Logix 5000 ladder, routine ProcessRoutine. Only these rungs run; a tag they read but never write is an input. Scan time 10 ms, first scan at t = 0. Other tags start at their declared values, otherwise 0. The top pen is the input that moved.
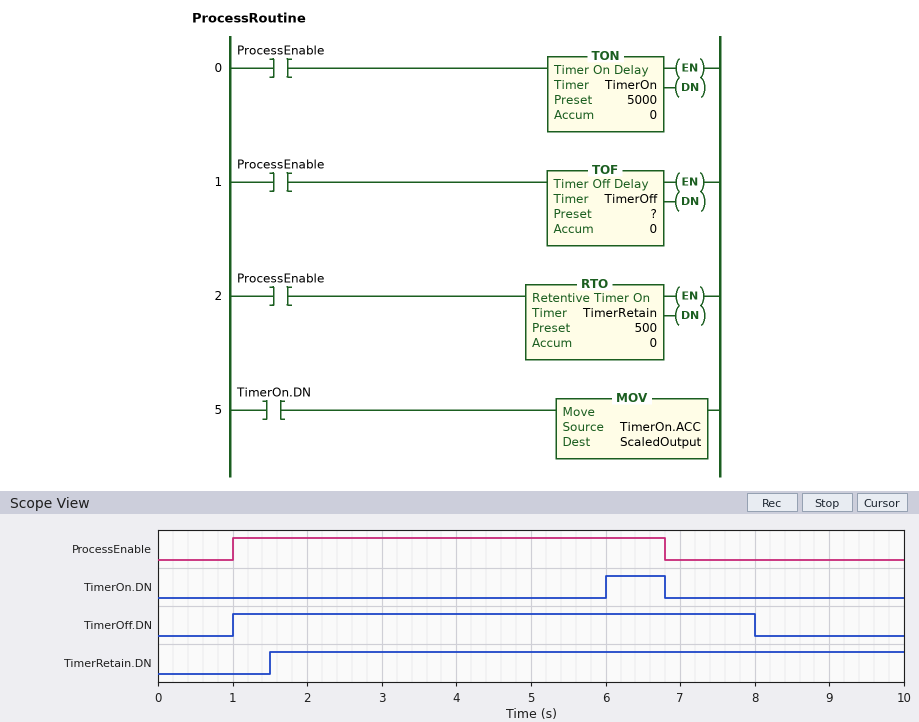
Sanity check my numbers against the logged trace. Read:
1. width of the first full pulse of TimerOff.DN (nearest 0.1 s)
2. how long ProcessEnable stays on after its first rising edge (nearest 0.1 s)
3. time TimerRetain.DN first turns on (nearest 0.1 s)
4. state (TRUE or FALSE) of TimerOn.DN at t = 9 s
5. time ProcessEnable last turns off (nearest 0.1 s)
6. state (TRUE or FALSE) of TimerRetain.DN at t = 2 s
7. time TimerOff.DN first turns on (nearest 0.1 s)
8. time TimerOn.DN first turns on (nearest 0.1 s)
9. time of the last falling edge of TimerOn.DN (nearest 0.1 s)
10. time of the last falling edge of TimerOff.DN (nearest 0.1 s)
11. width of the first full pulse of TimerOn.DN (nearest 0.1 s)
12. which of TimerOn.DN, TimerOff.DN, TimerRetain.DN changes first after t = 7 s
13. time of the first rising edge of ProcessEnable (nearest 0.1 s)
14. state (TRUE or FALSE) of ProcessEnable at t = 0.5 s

7.0 s
5.8 s
1.5 s
FALSE
6.8 s
TRUE
1.0 s
6.0 s
6.8 s
8.0 s
0.8 s
TimerOff.DN
1.0 s
FALSE
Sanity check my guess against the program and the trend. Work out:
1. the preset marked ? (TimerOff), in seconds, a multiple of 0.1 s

1.2 s
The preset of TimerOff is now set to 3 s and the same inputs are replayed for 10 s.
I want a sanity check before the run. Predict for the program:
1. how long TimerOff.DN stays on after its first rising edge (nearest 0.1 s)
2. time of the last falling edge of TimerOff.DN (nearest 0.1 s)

8.8 s
9.8 s
